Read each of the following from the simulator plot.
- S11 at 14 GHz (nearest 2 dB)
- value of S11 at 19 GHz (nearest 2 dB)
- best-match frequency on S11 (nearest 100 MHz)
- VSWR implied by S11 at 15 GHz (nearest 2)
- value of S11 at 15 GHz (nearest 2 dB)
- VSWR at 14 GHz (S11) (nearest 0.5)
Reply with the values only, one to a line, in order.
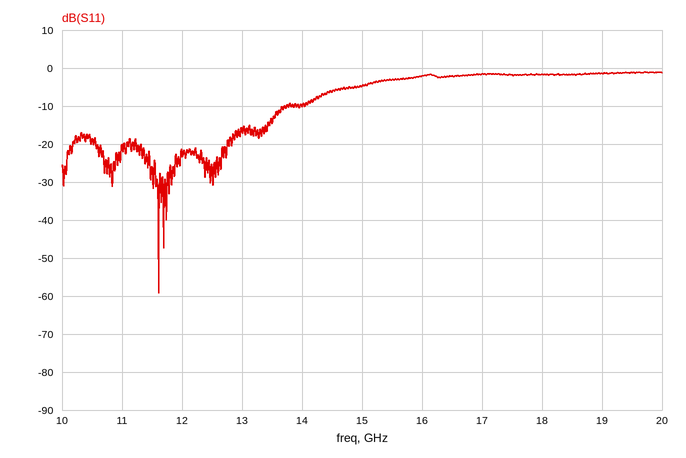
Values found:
-10 dB
-2 dB
11.6 GHz
4
-4 dB
2.0
